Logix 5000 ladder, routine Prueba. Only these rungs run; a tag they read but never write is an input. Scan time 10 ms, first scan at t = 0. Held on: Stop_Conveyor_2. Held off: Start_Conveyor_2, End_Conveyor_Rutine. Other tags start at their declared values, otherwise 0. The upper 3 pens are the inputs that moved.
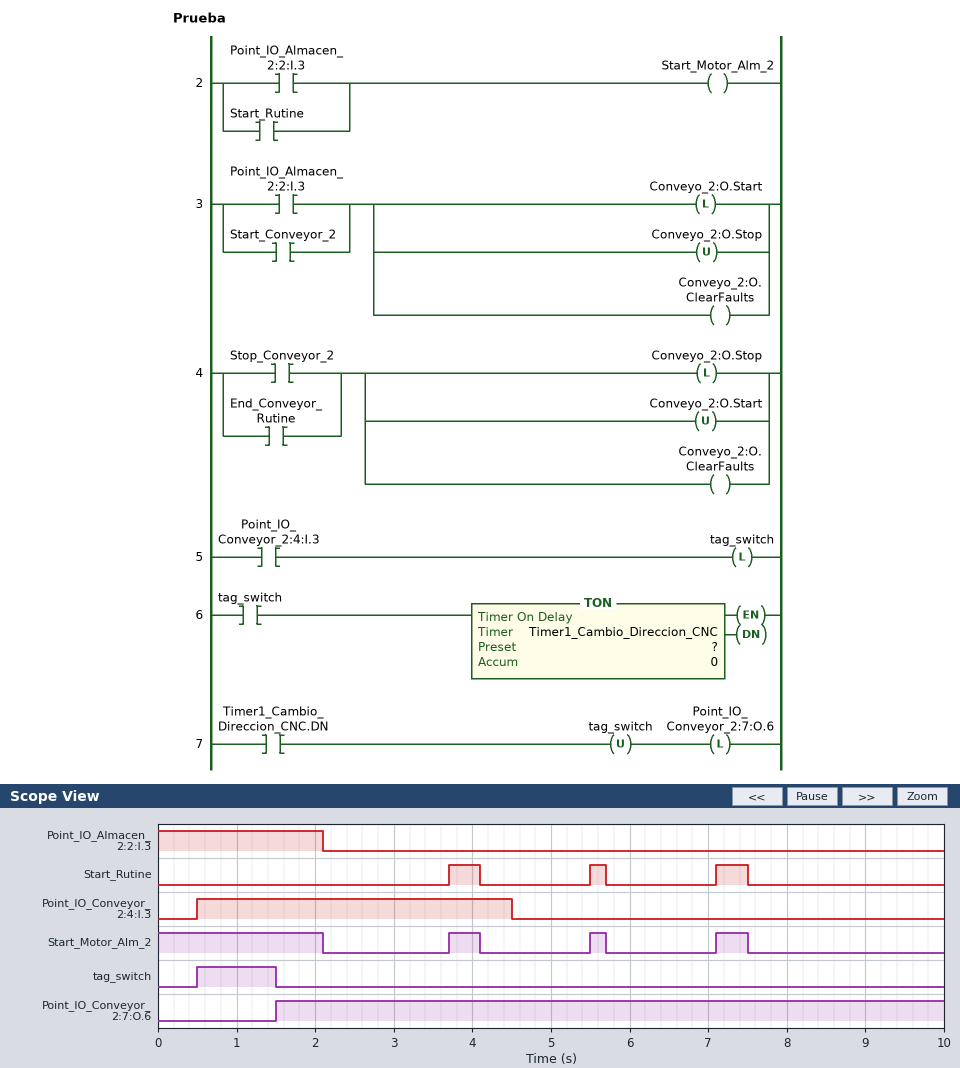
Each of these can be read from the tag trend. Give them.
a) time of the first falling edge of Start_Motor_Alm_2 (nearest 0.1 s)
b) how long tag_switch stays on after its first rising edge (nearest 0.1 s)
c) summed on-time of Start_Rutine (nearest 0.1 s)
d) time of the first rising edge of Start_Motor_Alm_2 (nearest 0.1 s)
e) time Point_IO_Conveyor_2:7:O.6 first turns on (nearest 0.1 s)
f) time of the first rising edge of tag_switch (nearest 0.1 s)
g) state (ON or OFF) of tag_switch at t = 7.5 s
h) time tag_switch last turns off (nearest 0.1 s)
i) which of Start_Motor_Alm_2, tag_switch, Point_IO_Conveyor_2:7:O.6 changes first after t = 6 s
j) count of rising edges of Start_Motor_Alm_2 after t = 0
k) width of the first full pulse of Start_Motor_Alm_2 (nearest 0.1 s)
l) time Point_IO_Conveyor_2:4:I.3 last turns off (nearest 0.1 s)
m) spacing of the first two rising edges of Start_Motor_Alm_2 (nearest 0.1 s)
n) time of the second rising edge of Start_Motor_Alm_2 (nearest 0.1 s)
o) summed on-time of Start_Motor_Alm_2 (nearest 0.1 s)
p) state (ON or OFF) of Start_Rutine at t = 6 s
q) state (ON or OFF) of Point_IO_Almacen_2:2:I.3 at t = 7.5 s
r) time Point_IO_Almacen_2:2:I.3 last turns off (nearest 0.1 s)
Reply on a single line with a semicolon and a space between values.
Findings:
2.1 s; 1.0 s; 1.0 s; 3.7 s; 1.5 s; 0.5 s; OFF; 1.5 s; Start_Motor_Alm_2; 3; 0.4 s; 4.5 s; 1.8 s; 5.5 s; 3.1 s; OFF; OFF; 2.1 s
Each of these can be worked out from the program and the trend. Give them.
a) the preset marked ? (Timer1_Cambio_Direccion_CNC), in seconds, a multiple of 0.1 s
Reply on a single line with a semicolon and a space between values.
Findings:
1.0 s
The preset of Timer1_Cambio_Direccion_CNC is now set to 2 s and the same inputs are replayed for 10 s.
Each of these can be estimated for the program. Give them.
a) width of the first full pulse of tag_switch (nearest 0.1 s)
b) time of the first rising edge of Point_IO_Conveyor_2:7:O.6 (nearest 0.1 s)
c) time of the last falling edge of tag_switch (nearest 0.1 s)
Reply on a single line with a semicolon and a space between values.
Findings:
2.0 s; 2.5 s; 2.5 s
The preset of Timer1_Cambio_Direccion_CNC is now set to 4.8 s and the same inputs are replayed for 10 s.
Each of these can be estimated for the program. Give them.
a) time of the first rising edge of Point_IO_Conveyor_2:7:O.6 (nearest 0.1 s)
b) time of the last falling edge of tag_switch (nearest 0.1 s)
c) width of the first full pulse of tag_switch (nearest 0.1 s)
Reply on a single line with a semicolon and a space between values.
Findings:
5.3 s; 5.3 s; 4.8 s
